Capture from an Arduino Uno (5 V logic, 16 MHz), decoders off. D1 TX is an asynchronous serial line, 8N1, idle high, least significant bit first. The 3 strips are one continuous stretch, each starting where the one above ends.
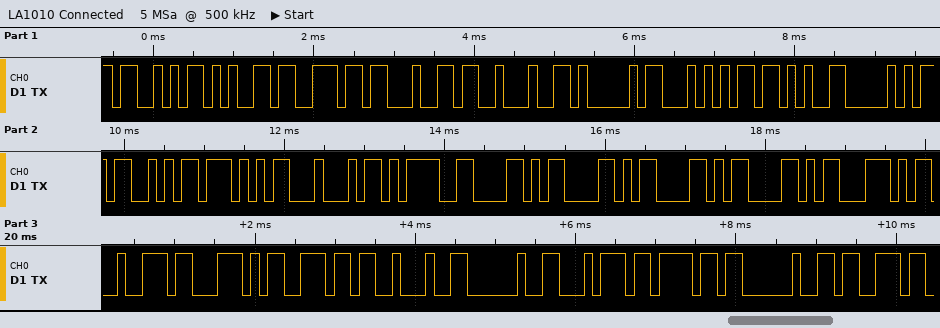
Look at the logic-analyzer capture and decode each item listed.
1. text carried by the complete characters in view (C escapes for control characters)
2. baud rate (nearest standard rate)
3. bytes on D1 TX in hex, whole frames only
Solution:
"Send\"AT+PSWD=XXXX\\r\\n\" to s"
9600 baud
53 65 6E 64 22 41 54 2B 50 53 57 44 3D 58 58 58 58 5C 72 5C 6E 22 20 74 6F 20 73
